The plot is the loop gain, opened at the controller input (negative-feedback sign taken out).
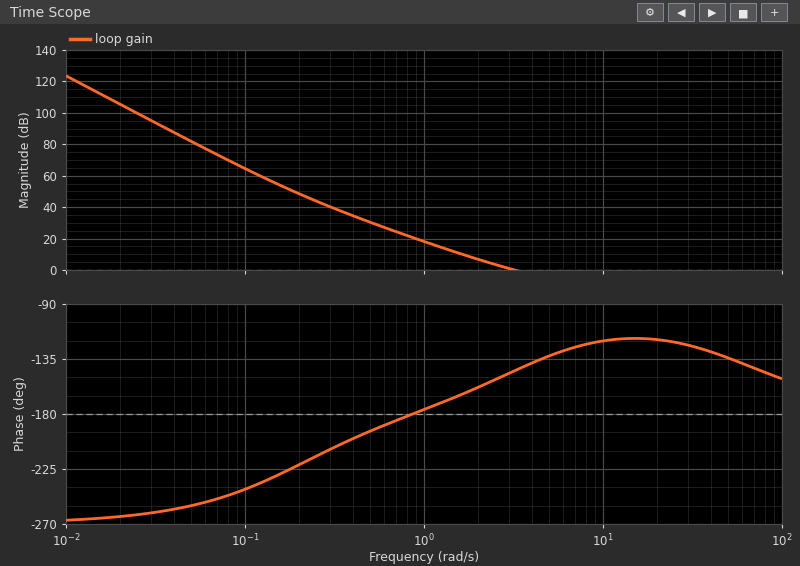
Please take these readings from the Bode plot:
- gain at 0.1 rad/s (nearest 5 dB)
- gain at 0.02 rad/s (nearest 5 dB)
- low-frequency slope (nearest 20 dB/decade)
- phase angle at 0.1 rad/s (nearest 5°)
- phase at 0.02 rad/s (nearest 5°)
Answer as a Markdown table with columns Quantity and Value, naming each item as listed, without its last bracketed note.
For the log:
| Quantity | Value |
|---|---|
| gain at 0.1 rad/s | 65 dB |
| gain at 0.02 rad/s | 105 dB |
| low-frequency slope | -60 dB/decade |
| phase angle at 0.1 rad/s | -240° |
| phase at 0.02 rad/s | -265° |
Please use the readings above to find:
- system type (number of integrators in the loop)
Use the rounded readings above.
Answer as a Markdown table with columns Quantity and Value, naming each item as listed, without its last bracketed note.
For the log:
| Quantity | Value |
|---|---|
| system type | 3 |
